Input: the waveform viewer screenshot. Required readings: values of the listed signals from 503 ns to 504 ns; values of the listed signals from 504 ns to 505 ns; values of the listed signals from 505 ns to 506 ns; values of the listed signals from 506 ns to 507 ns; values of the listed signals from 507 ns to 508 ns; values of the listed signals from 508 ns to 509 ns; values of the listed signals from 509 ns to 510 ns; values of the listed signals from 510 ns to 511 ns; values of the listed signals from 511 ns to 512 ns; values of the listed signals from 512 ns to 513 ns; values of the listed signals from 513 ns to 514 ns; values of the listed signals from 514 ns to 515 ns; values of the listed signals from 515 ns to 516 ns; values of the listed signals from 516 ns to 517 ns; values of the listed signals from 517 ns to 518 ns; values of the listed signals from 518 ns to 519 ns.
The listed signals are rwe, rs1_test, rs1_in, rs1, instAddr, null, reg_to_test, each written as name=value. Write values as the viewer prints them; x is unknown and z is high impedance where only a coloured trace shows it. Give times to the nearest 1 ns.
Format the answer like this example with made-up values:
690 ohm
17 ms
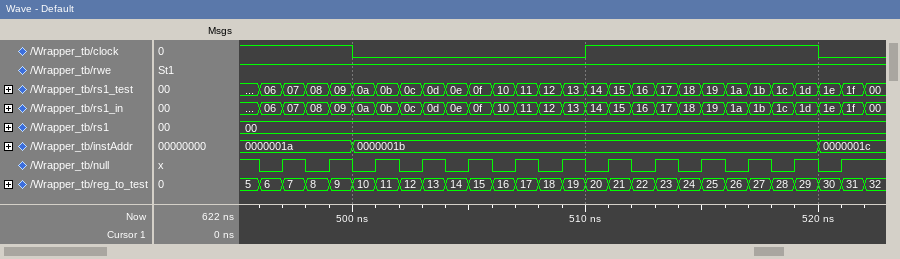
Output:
rwe=1, rs1_test=0d, rs1_in=0d, rs1=00, instAddr=0000001b, null=1, reg_to_test=13
rwe=1, rs1_test=0e, rs1_in=0e, rs1=00, instAddr=0000001b, null=0, reg_to_test=14
rwe=1, rs1_test=0f, rs1_in=0f, rs1=00, instAddr=0000001b, null=1, reg_to_test=15
rwe=1, rs1_test=10, rs1_in=10, rs1=00, instAddr=0000001b, null=0, reg_to_test=16
rwe=1, rs1_test=11, rs1_in=11, rs1=00, instAddr=0000001b, null=1, reg_to_test=17
rwe=1, rs1_test=12, rs1_in=12, rs1=00, instAddr=0000001b, null=0, reg_to_test=18
rwe=1, rs1_test=13, rs1_in=13, rs1=00, instAddr=0000001b, null=1, reg_to_test=19
rwe=1, rs1_test=14, rs1_in=14, rs1=00, instAddr=0000001b, null=0, reg_to_test=20
rwe=1, rs1_test=15, rs1_in=15, rs1=00, instAddr=0000001b, null=1, reg_to_test=21
rwe=1, rs1_test=16, rs1_in=16, rs1=00, instAddr=0000001b, null=0, reg_to_test=22
rwe=1, rs1_test=17, rs1_in=17, rs1=00, instAddr=0000001b, null=1, reg_to_test=23
rwe=1, rs1_test=18, rs1_in=18, rs1=00, instAddr=0000001b, null=0, reg_to_test=24
rwe=1, rs1_test=19, rs1_in=19, rs1=00, instAddr=0000001b, null=1, reg_to_test=25
rwe=1, rs1_test=1a, rs1_in=1a, rs1=00, instAddr=0000001b, null=0, reg_to_test=26
rwe=1, rs1_test=1b, rs1_in=1b, rs1=00, instAddr=0000001b, null=1, reg_to_test=27
rwe=1, rs1_test=1c, rs1_in=1c, rs1=00, instAddr=0000001b, null=0, reg_to_test=28
